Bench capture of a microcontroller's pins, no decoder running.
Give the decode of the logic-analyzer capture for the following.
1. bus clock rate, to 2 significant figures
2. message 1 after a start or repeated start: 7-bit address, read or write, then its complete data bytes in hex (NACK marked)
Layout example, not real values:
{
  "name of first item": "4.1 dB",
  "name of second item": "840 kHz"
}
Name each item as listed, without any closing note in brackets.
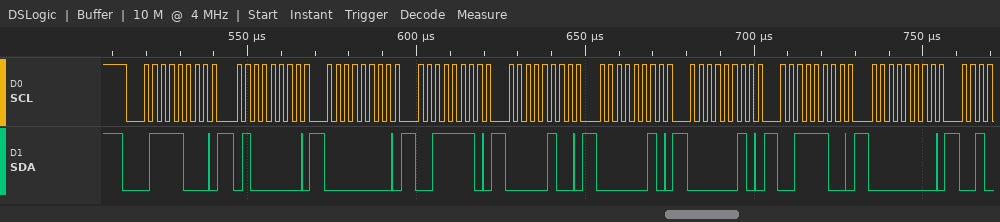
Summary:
{
  "bus clock rate, to 2 significant figures": "400 kHz",
  "message 1 after a start or repeated start: 7-bit address, read or write, then its complete data bytes in hex": "0x3C write: 40 00 3E 04 02 02 3C 00"
}
